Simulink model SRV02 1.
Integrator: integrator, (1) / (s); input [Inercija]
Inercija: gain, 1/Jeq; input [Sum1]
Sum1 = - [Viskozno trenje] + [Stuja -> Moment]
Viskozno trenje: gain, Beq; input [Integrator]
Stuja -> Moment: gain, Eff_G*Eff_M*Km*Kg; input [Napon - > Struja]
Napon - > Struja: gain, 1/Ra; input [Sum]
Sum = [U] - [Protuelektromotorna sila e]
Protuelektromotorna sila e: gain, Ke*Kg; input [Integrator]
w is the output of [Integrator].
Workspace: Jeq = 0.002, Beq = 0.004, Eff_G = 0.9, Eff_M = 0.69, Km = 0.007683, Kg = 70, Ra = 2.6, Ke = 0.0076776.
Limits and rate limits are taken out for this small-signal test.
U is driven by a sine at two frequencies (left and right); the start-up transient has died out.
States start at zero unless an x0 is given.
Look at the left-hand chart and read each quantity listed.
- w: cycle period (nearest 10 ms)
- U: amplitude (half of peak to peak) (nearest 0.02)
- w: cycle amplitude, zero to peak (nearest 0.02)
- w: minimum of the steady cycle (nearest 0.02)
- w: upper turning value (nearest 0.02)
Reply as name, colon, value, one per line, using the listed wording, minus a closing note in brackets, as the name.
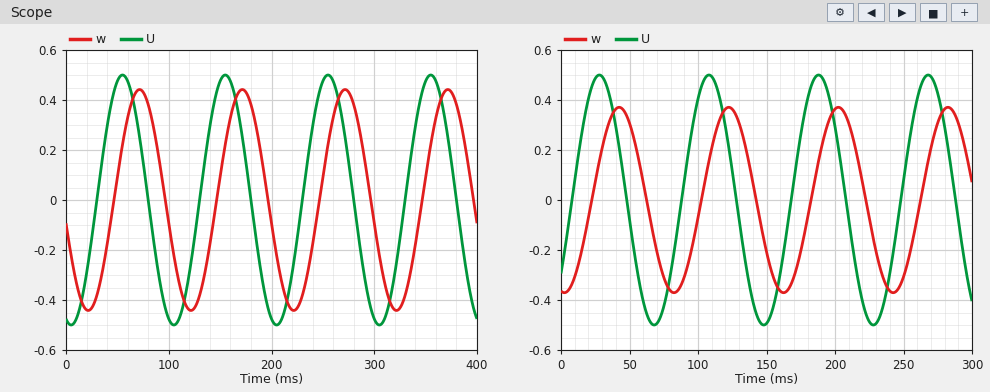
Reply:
w: cycle period: 100 ms
U: amplitude (half of peak to peak): 0.50
w: cycle amplitude, zero to peak: 0.44
w: minimum of the steady cycle: -0.44
w: upper turning value: 0.44
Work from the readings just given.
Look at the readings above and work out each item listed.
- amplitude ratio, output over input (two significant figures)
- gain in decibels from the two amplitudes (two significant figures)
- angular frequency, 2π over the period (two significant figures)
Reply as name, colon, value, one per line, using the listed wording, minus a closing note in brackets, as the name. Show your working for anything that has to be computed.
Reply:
amplitude ratio, output over input: 0.44 / 0.5 = 0.88
gain in decibels from the two amplitudes: 20 log10(0.44 / 0.5) = -1.1 dB
angular frequency, 2π over the period: 2π / 100 = 0.063 rad/ms
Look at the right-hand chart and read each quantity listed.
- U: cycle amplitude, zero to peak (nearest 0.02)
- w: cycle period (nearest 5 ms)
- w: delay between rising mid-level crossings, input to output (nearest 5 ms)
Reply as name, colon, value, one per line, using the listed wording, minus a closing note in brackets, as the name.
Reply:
U: cycle amplitude, zero to peak: 0.50
w: cycle period: 80 ms
w: delay between rising mid-level crossings, input to output: 15 ms
